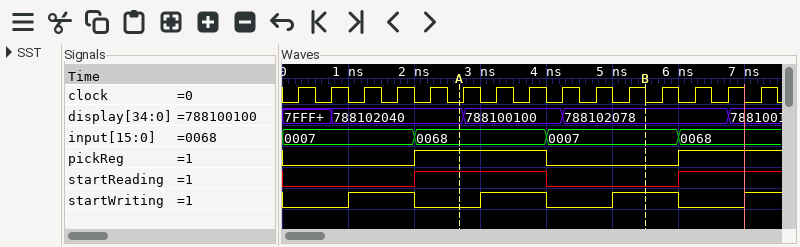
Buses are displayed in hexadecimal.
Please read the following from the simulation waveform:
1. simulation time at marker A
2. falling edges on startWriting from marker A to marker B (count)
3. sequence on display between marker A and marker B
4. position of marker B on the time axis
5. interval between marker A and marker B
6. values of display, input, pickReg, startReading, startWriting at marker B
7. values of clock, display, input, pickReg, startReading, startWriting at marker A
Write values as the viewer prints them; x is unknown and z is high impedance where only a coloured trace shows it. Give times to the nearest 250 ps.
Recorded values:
2750 ps
1
788102040, 788100100, 788102078
5500 ps
2750 ps
display=788102078, input=0007, pickReg=0, startReading=0, startWriting=1
clock=0, display=788102040, input=0068, pickReg=1, startReading=1, startWriting=0
